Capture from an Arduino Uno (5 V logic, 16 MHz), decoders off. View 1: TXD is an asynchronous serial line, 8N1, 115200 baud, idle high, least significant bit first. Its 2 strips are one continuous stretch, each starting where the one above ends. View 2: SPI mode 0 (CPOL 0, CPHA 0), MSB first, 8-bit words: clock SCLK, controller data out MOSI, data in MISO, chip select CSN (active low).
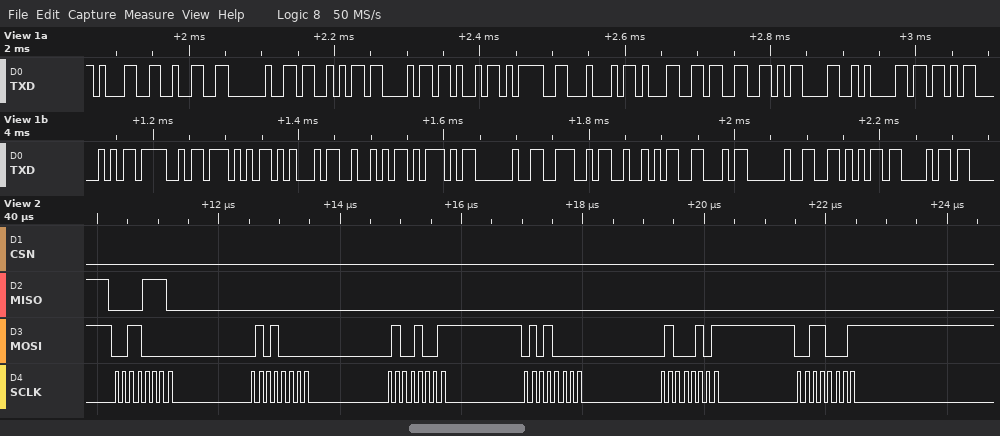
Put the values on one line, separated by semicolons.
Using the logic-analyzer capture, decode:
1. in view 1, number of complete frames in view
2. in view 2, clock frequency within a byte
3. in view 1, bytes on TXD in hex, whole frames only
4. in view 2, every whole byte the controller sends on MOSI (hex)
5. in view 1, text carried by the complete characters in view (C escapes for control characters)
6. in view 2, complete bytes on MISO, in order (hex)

26; 8 MHz; 0x31 0x32 0x20 0x53 0x43 0x4B 0x3D 0x44 0x31 0x33 0x0D 0x0A 0x5B 0x50 0x4F 0x57 0x45 0x52 0x5D 0x20 0x4E 0x52 0x46 0x20 0x56 0x43; 0x30 0x50 0x49 0x50 0x45 0x31; "12 SCK=D13\r\n[POWER] NRF VC"; 0x0E 0x00 0x00 0x00 0x00 0x00
